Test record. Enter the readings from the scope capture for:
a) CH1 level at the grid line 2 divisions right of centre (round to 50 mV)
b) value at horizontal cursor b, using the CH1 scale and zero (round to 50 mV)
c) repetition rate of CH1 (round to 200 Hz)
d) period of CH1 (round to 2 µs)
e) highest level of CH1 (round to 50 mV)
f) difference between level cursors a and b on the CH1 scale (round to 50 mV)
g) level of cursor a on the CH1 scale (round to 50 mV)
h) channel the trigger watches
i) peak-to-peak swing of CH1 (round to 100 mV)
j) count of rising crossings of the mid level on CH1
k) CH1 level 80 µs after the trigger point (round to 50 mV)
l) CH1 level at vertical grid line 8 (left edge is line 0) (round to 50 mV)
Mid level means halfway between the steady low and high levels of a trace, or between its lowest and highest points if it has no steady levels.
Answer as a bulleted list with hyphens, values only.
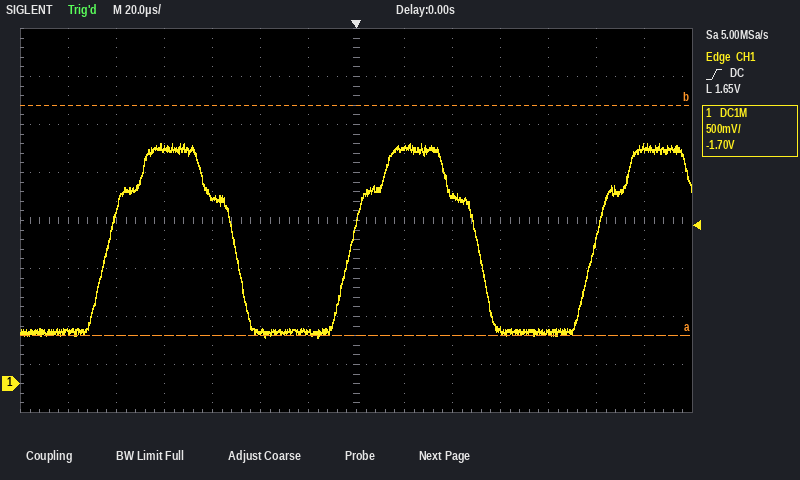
- 1.95 V
- 2.90 V
- 9.8 kHz
- 102 µs
- 2.50 V
- 2.40 V
- 500 mV
- CH1
- 2.00 V
- 3
- 550 mV
- 2.45 V
